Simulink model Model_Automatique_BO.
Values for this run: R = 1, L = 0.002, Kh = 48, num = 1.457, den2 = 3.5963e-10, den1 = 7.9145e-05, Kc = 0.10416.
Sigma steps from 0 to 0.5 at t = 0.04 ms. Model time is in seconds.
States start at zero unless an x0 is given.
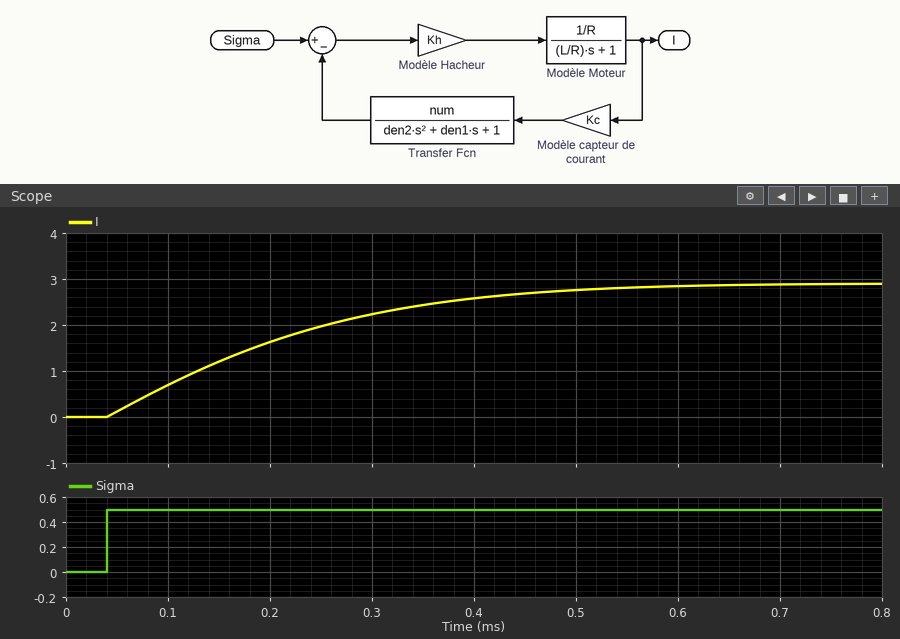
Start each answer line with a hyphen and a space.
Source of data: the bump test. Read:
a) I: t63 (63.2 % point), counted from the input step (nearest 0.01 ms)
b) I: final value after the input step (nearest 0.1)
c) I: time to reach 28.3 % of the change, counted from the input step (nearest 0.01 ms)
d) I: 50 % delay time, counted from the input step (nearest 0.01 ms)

- 0.19 ms
- 2.9
- 0.07 ms
- 0.14 ms
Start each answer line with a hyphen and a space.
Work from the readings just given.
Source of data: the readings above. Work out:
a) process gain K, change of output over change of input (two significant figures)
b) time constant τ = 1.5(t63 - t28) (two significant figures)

- 5.8
- 0.18 ms
